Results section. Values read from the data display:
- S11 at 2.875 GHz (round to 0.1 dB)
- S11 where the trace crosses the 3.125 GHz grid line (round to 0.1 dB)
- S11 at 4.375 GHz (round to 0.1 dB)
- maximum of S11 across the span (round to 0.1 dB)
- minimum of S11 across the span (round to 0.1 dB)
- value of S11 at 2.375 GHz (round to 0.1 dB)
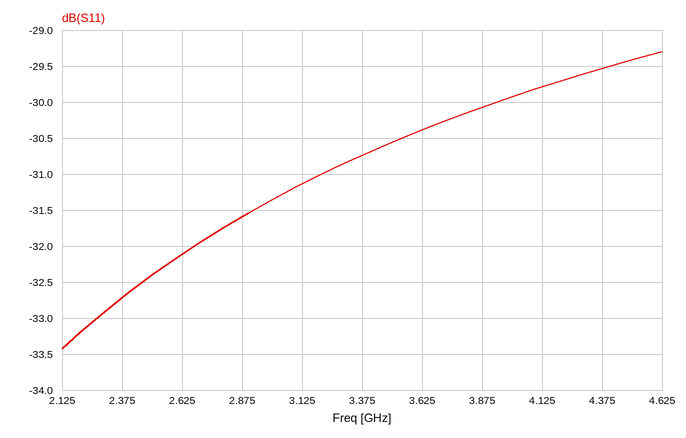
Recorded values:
-31.6 dB
-31.1 dB
-29.5 dB
-29.3 dB
-33.4 dB
-32.7 dB
